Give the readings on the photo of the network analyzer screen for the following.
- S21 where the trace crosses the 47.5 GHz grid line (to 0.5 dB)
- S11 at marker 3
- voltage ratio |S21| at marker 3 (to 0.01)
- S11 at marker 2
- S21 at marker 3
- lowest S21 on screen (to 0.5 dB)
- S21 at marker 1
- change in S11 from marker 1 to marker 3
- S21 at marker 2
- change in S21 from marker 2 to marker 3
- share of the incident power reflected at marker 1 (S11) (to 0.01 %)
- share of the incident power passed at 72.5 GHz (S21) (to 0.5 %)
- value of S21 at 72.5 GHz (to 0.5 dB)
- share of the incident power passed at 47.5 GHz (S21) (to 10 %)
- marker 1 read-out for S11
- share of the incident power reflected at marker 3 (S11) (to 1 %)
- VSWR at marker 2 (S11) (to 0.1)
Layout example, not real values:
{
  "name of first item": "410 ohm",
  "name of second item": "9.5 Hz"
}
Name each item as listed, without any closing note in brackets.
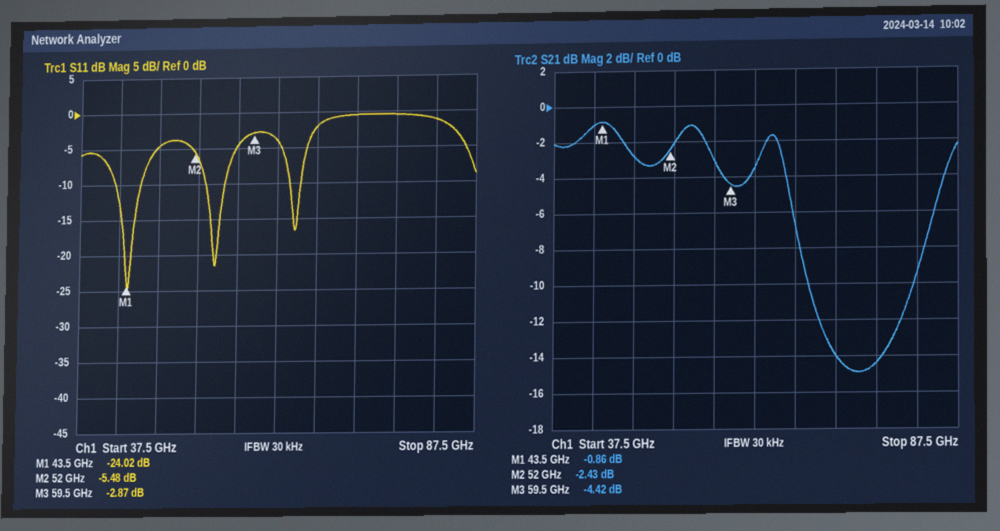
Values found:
{
  "S21 where the trace crosses the 47.5 GHz grid line": "-3.0 dB",
  "S11 at marker 3": "-2.87 dB",
  "voltage ratio |S21| at marker 3": "0.60",
  "S11 at marker 2": "-5.48 dB",
  "S21 at marker 3": "-4.42 dB",
  "lowest S21 on screen": "-15.0 dB",
  "S21 at marker 1": "-0.86 dB",
  "change in S11 from marker 1 to marker 3": "21.15 dB",
  "S21 at marker 2": "-2.43 dB",
  "change in S21 from marker 2 to marker 3": "-1.99 dB",
  "share of the incident power reflected at marker 1 (S11)": "0.40 %",
  "share of the incident power passed at 72.5 GHz (S21)": "4.0 %",
  "value of S21 at 72.5 GHz": "-14.0 dB",
  "share of the incident power passed at 47.5 GHz (S21)": "50 %",
  "marker 1 read-out for S11": "-24.02 dB",
  "share of the incident power reflected at marker 3 (S11)": "52 %",
  "VSWR at marker 2 (S11)": "3.3"
}
